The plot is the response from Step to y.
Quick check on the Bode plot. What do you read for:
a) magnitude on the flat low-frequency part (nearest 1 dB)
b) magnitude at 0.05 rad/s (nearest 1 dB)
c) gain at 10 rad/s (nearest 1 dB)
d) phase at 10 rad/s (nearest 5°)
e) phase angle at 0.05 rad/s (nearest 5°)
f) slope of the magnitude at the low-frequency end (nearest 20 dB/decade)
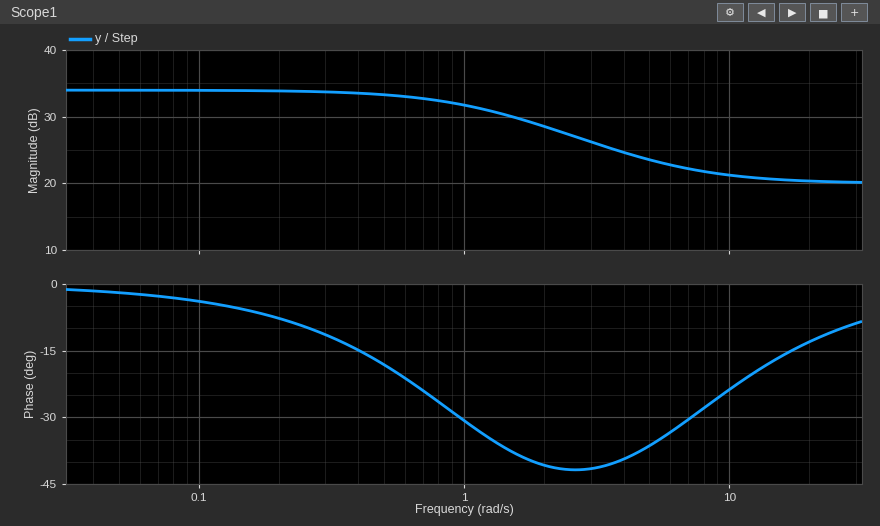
34 dB
34 dB
21 dB
-25°
0°
0 dB/decade
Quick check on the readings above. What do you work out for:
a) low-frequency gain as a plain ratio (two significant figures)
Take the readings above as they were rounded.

50
